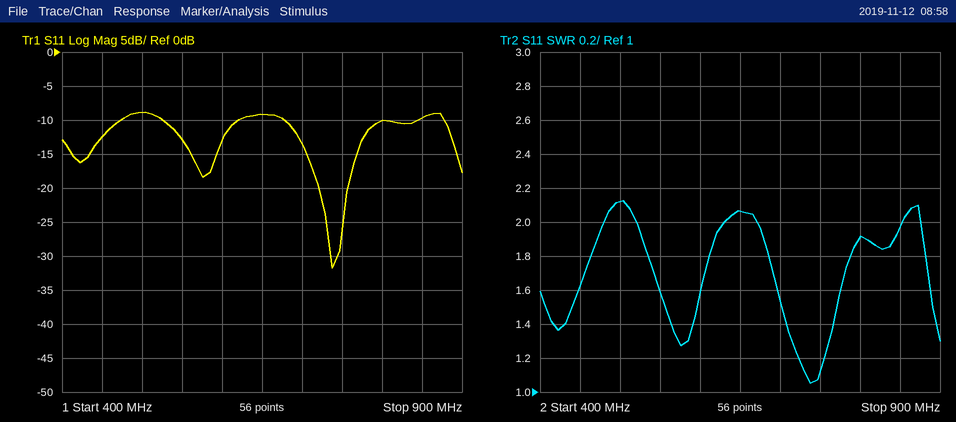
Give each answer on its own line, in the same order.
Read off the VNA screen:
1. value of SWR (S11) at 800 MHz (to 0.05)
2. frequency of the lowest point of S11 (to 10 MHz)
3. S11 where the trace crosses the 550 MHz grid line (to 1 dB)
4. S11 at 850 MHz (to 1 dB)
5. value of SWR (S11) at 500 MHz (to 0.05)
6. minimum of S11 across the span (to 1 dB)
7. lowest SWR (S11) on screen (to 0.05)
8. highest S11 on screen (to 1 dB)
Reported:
1.90
740 MHz
-13 dB
-10 dB
2.10
-32 dB
1.05
-9 dB
